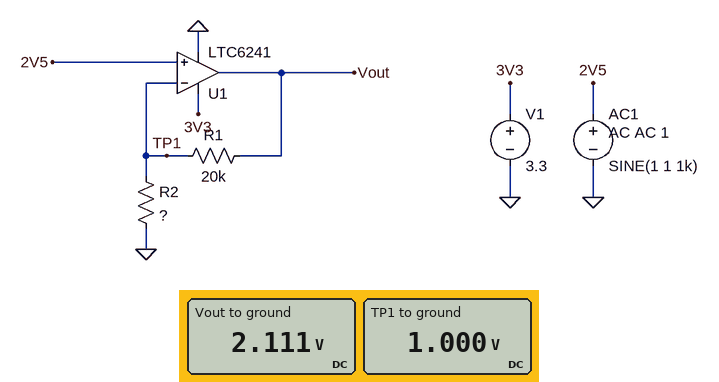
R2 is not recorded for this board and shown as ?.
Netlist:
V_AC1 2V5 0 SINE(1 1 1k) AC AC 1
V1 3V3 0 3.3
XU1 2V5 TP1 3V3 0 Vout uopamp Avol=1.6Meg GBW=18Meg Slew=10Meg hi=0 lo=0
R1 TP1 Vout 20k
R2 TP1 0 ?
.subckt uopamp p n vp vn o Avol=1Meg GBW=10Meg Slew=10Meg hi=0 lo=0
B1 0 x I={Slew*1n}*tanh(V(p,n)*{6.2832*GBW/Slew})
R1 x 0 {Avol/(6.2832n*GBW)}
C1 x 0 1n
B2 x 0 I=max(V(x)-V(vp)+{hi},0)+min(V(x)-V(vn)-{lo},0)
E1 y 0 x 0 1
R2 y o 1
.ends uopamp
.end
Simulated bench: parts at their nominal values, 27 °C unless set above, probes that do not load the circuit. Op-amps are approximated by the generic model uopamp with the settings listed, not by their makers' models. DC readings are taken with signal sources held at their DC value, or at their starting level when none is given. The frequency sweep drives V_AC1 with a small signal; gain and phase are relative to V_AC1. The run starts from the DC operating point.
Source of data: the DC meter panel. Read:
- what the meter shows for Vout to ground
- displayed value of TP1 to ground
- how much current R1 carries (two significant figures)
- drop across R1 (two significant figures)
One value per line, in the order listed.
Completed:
2.111 V
1.000 V
56 µA
1.1 V
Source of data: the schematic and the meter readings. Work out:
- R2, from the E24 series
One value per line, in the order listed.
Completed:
18 kΩ
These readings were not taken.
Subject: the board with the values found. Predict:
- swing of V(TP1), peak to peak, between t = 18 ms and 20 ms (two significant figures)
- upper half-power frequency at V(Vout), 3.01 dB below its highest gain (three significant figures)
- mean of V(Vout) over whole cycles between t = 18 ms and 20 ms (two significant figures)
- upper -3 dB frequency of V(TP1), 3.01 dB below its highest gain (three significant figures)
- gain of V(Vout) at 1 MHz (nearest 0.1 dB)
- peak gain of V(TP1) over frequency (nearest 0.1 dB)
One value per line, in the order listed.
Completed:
1.6 V
8.53 MHz
1.9 V
8.53 MHz
6.4 dB
0 dB
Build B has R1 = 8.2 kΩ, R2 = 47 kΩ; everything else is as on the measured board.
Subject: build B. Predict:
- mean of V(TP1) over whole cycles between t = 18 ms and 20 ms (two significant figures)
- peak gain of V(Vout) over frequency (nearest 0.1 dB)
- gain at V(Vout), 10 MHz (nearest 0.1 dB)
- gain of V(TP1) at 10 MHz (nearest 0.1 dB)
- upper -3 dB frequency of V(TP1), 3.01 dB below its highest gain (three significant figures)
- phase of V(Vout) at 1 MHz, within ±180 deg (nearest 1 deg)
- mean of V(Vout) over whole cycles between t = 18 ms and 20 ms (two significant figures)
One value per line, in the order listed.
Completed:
1.0 V
1.4 dB
-0.1 dB
-1.5 dB
15.3 MHz
-4 deg
1.2 V
